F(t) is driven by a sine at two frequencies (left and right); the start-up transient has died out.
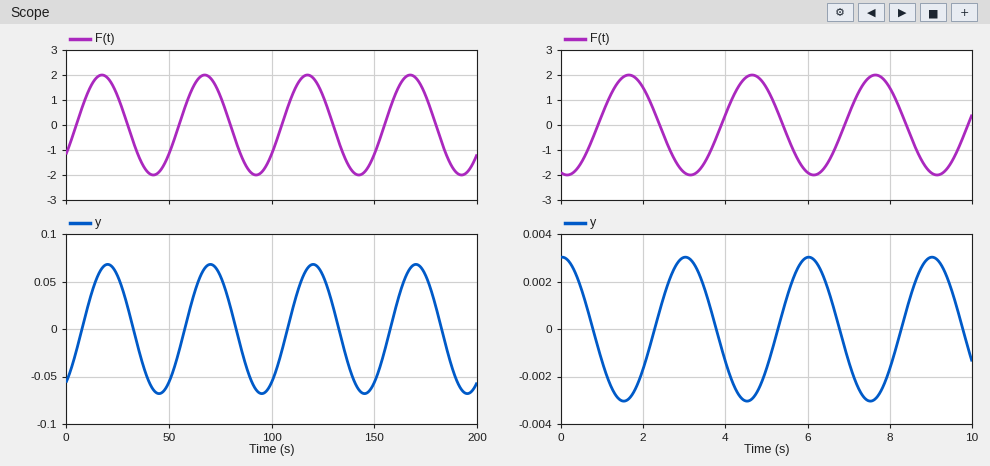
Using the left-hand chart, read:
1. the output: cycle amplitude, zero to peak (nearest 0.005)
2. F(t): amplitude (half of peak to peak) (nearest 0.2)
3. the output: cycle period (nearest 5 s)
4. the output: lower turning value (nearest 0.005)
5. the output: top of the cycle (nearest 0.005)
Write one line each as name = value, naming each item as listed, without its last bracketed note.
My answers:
the output: cycle amplitude, zero to peak = 0.070
F(t): amplitude (half of peak to peak) = 2.0
the output: cycle period = 50 s
the output: lower turning value = -0.070
the output: top of the cycle = 0.070
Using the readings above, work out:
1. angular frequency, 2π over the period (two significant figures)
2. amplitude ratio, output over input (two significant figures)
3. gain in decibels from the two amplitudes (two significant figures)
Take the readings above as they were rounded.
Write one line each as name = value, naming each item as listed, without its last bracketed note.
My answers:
angular frequency, 2π over the period = 0.13 rad/s
amplitude ratio, output over input = 0.035
gain in decibels from the two amplitudes = -29 dB
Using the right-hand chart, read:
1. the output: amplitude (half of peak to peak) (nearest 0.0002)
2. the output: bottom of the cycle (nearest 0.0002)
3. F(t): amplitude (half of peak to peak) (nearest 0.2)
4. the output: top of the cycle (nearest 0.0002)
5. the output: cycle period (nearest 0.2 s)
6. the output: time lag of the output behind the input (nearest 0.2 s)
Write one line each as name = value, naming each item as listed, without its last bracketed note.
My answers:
the output: amplitude (half of peak to peak) = 0.0030
the output: bottom of the cycle = -0.0030
F(t): amplitude (half of peak to peak) = 2.0
the output: top of the cycle = 0.0030
the output: cycle period = 3.0 s
the output: time lag of the output behind the input = 1.4 s
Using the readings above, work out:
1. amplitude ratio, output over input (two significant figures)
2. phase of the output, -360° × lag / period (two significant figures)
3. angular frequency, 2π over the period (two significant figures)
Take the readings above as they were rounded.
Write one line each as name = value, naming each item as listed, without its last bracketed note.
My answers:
amplitude ratio, output over input = 0.0015
phase of the output, -360° × lag / period = -170°
angular frequency, 2π over the period = 2.1 rad/s
